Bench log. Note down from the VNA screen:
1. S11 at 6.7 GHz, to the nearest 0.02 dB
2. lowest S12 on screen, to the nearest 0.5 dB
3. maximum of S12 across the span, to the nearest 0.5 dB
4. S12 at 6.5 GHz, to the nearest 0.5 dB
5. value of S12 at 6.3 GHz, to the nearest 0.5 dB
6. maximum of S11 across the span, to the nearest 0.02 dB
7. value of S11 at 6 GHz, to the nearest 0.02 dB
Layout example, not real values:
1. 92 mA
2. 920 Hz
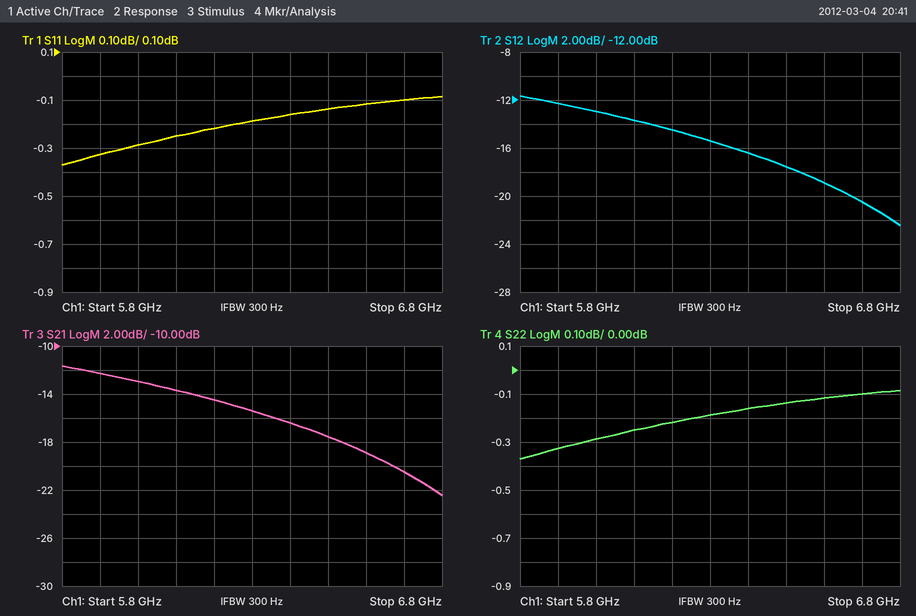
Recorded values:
1. -0.10 dB
2. -22.5 dB
3. -11.5 dB
4. -17.5 dB
5. -15.5 dB
6. -0.08 dB
7. -0.28 dB
